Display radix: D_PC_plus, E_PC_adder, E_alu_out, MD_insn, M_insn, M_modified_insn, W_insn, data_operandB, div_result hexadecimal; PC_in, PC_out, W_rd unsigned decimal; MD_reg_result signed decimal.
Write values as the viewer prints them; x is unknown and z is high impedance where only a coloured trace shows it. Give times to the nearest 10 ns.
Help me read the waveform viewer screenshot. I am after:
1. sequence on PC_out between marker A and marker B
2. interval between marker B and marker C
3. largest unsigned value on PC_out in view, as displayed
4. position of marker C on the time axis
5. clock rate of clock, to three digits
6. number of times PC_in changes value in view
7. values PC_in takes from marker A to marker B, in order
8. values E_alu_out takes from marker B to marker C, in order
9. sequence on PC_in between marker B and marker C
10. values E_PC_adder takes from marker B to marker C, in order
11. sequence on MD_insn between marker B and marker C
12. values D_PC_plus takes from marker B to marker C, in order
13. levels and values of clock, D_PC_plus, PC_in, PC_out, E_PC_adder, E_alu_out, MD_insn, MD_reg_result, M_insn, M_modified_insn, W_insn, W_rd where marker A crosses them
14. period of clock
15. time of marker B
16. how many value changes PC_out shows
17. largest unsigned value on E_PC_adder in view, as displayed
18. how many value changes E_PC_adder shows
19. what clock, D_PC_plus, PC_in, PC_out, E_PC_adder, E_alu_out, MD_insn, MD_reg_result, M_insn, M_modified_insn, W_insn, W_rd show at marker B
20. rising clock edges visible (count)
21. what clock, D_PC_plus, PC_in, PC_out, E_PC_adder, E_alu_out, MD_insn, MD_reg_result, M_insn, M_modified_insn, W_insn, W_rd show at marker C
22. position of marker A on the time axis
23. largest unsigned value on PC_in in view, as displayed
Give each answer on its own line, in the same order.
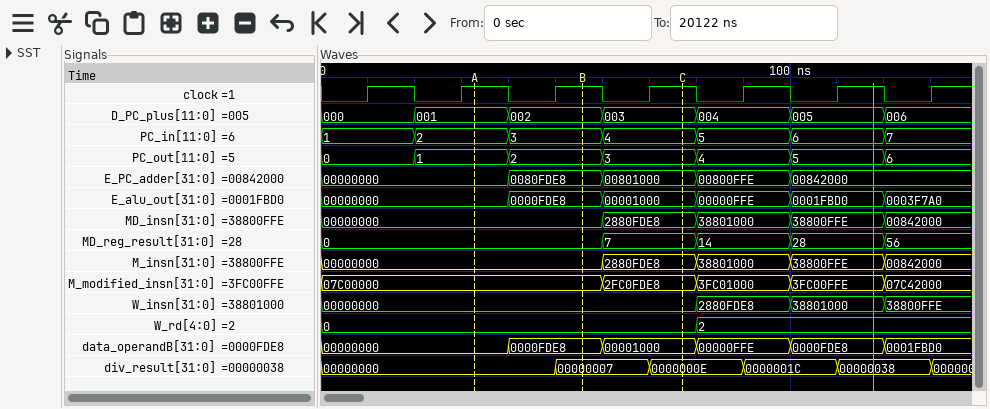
1, 2
20 ns
6
80 ns
50.0 MHz
6
2, 3
0000FDE8, 00001000
3, 4
0080FDE8, 00801000
00000000, 2880FDE8
002, 003
clock=1, D_PC_plus=001, PC_in=2, PC_out=1, E_PC_adder=00000000, E_alu_out=00000000, MD_insn=00000000, MD_reg_result=0, M_insn=00000000, M_modified_insn=07C00000, W_insn=00000000, W_rd=0
20 ns
60 ns
6
00842000
4
clock=1, D_PC_plus=002, PC_in=3, PC_out=2, E_PC_adder=0080FDE8, E_alu_out=0000FDE8, MD_insn=00000000, MD_reg_result=0, M_insn=00000000, M_modified_insn=07C00000, W_insn=00000000, W_rd=0
7
clock=1, D_PC_plus=003, PC_in=4, PC_out=3, E_PC_adder=00801000, E_alu_out=00001000, MD_insn=2880FDE8, MD_reg_result=7, M_insn=2880FDE8, M_modified_insn=2FC0FDE8, W_insn=00000000, W_rd=0
30 ns
7
